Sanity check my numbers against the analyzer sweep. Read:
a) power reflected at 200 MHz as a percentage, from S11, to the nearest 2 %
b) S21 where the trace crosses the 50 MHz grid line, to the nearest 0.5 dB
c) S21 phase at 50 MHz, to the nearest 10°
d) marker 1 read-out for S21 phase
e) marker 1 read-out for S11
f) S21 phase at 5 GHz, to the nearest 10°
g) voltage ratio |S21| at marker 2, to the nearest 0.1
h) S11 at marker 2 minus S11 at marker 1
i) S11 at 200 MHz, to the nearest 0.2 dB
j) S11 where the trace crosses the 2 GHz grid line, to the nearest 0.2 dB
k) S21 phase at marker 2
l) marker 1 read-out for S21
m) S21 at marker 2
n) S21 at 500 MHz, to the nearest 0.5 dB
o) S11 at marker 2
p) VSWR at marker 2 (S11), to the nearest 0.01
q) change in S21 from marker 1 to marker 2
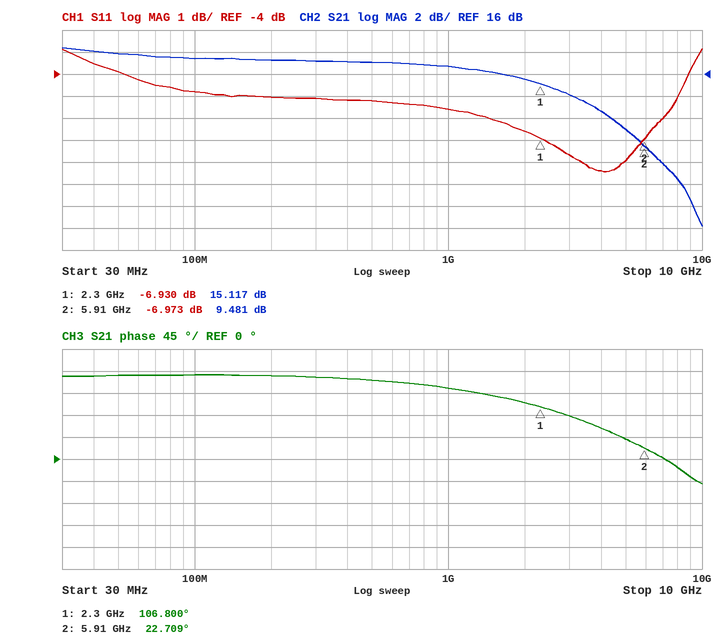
32 %
18.0 dB
170°
106.800°
-6.930 dB
40°
3.0
-0.043 dB
-5.0 dB
-6.6 dB
22.709°
15.117 dB
9.481 dB
17.0 dB
-6.973 dB
2.62
-5.636 dB
